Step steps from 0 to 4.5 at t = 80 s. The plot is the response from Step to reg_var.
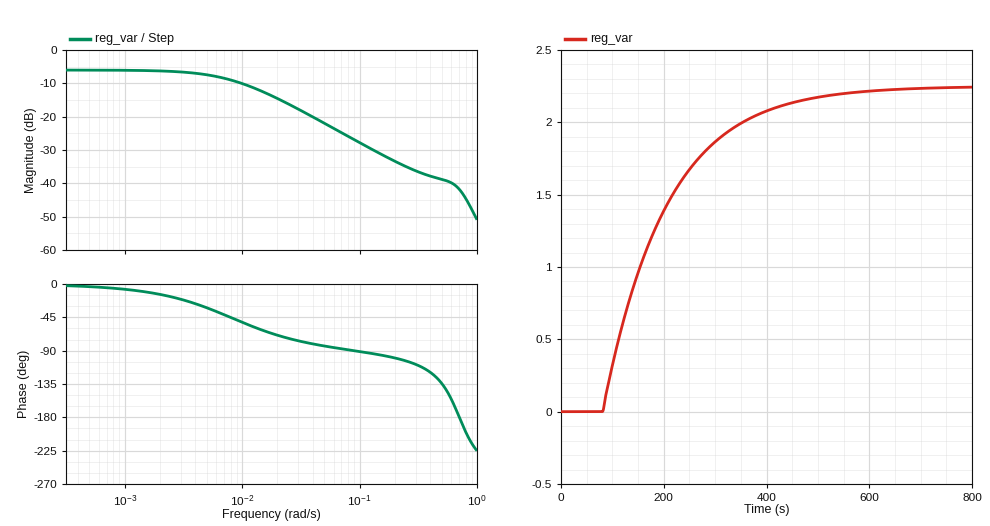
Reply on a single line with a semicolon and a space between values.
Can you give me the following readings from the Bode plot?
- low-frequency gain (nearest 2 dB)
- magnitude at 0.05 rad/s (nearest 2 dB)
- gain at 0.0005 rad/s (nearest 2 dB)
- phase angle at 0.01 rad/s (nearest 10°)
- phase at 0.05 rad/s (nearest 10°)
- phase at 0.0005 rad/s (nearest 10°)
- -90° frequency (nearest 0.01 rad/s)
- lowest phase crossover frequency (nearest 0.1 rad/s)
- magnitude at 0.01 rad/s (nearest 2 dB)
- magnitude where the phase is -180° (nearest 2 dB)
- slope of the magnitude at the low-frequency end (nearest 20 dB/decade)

-6 dB; -22 dB; -6 dB; -50°; -80°; 0°; 0.09 rad/s; 0.7 rad/s; -10 dB; -42 dB; 0 dB/decade
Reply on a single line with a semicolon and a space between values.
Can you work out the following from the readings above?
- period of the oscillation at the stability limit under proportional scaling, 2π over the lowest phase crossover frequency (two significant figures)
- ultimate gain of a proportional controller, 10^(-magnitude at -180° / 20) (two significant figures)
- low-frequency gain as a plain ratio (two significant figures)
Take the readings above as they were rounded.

9.0 s; 130; 0.50
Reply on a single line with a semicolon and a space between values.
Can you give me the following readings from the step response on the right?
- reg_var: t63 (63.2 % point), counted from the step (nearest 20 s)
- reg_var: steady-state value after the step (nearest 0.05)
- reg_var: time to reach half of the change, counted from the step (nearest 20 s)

120 s; 2.25; 80 s
